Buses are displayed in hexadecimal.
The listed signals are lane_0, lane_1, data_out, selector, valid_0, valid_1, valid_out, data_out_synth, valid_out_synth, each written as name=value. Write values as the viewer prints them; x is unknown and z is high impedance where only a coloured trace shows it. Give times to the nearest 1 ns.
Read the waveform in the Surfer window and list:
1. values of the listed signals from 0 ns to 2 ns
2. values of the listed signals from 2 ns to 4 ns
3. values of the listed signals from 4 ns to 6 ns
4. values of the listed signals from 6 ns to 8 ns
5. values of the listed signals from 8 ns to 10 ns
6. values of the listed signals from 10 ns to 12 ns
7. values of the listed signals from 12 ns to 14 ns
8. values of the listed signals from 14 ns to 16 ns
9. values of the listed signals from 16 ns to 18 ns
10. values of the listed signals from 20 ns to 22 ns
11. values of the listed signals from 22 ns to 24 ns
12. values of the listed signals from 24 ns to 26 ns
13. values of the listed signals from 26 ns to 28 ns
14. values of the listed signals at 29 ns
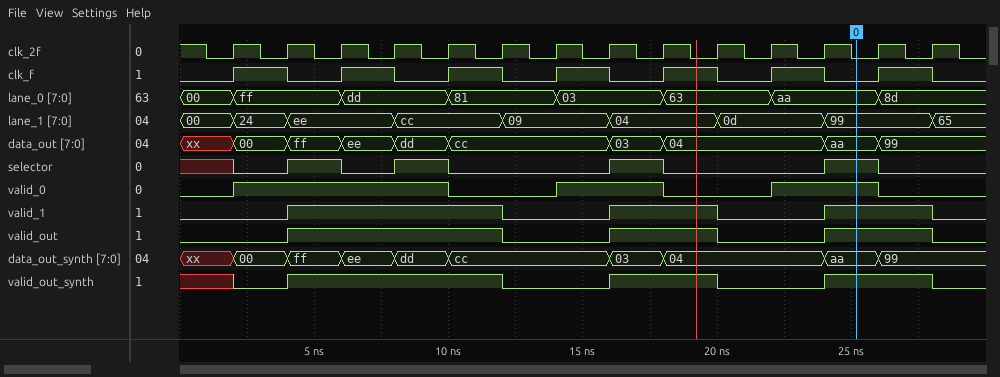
lane_0=00, lane_1=00, data_out=xx, selector=x, valid_0=0, valid_1=0, valid_out=0, data_out_synth=xx, valid_out_synth=x
lane_0=ff, lane_1=24, data_out=00, selector=0, valid_0=1, valid_1=0, valid_out=0, data_out_synth=00, valid_out_synth=0
lane_0=ff, lane_1=ee, data_out=ff, selector=1, valid_0=1, valid_1=1, valid_out=1, data_out_synth=ff, valid_out_synth=1
lane_0=dd, lane_1=ee, data_out=ee, selector=0, valid_0=1, valid_1=1, valid_out=1, data_out_synth=ee, valid_out_synth=1
lane_0=dd, lane_1=cc, data_out=dd, selector=1, valid_0=1, valid_1=1, valid_out=1, data_out_synth=dd, valid_out_synth=1
lane_0=81, lane_1=cc, data_out=cc, selector=0, valid_0=0, valid_1=1, valid_out=1, data_out_synth=cc, valid_out_synth=1
lane_0=81, lane_1=09, data_out=cc, selector=0, valid_0=0, valid_1=0, valid_out=0, data_out_synth=cc, valid_out_synth=0
lane_0=03, lane_1=09, data_out=cc, selector=0, valid_0=1, valid_1=0, valid_out=0, data_out_synth=cc, valid_out_synth=0
lane_0=03, lane_1=04, data_out=03, selector=1, valid_0=1, valid_1=1, valid_out=1, data_out_synth=03, valid_out_synth=1
lane_0=63, lane_1=0d, data_out=04, selector=0, valid_0=0, valid_1=0, valid_out=0, data_out_synth=04, valid_out_synth=0
lane_0=aa, lane_1=0d, data_out=04, selector=0, valid_0=1, valid_1=0, valid_out=0, data_out_synth=04, valid_out_synth=0
lane_0=aa, lane_1=99, data_out=aa, selector=1, valid_0=1, valid_1=1, valid_out=1, data_out_synth=aa, valid_out_synth=1
lane_0=8d, lane_1=99, data_out=99, selector=0, valid_0=0, valid_1=1, valid_out=1, data_out_synth=99, valid_out_synth=1
lane_0=8d, lane_1=65, data_out=99, selector=0, valid_0=0, valid_1=0, valid_out=0, data_out_synth=99, valid_out_synth=0
